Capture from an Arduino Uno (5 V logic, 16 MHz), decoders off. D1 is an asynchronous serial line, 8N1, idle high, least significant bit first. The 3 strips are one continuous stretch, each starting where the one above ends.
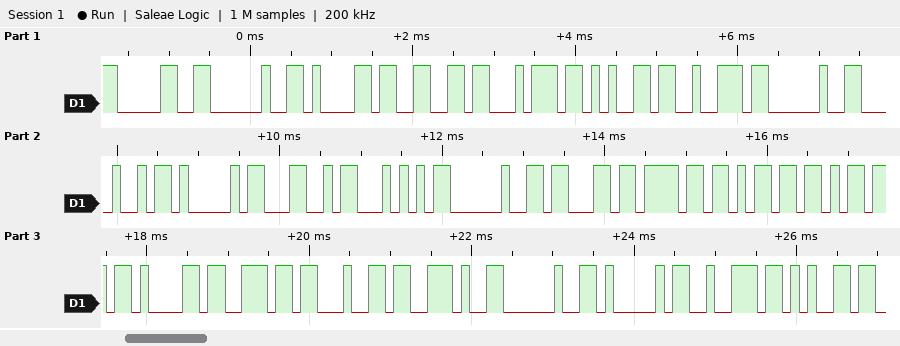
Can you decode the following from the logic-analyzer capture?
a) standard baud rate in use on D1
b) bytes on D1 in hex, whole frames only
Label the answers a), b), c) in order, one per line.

a) 9600 baud
b) 0x30 0x20 0x61 0x66 0x74 0x65 0x72 0x20 0x48 0x41 0x4C 0x54 0x20 0x63 0x6F 0x6D 0x6D 0x61 0x6E 0x64 0x2E 0x20 0x41 0x72 0x65
